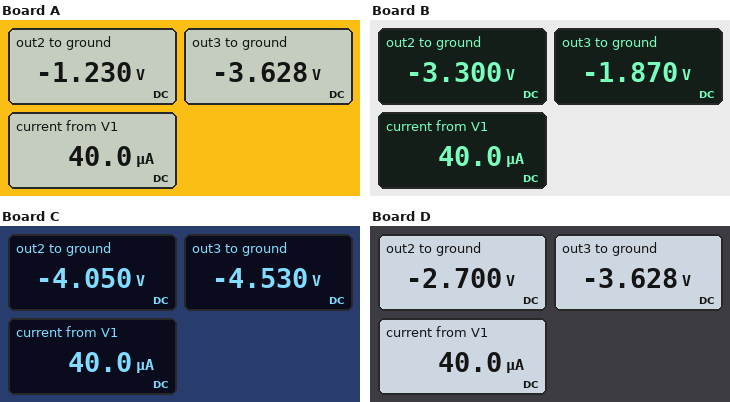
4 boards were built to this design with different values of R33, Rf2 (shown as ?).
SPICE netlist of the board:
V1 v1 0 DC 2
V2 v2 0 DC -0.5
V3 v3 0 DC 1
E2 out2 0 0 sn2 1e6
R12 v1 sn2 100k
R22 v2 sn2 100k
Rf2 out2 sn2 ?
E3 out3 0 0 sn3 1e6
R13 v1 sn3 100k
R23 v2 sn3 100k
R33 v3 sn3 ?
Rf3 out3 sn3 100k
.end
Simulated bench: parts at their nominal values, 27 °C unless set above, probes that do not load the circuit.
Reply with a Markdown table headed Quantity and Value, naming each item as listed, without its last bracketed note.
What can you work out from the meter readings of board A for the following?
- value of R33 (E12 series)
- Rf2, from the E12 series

| Quantity | Value |
|---|---|
| value of R33 | 47 kΩ |
| Rf2, from the E12 series | 82 kΩ |
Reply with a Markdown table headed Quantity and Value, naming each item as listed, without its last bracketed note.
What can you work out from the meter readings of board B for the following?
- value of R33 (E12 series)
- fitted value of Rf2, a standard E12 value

| Quantity | Value |
|---|---|
| value of R33 | 270 kΩ |
| fitted value of Rf2, a standard E12 value | 220 kΩ |
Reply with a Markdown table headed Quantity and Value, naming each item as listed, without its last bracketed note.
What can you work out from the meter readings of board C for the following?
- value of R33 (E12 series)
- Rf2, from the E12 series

| Quantity | Value |
|---|---|
| value of R33 | 33 kΩ |
| Rf2, from the E12 series | 270 kΩ |
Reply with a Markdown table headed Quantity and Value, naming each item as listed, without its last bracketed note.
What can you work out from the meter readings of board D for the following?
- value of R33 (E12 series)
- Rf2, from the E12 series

| Quantity | Value |
|---|---|
| value of R33 | 47 kΩ |
| Rf2, from the E12 series | 180 kΩ |
